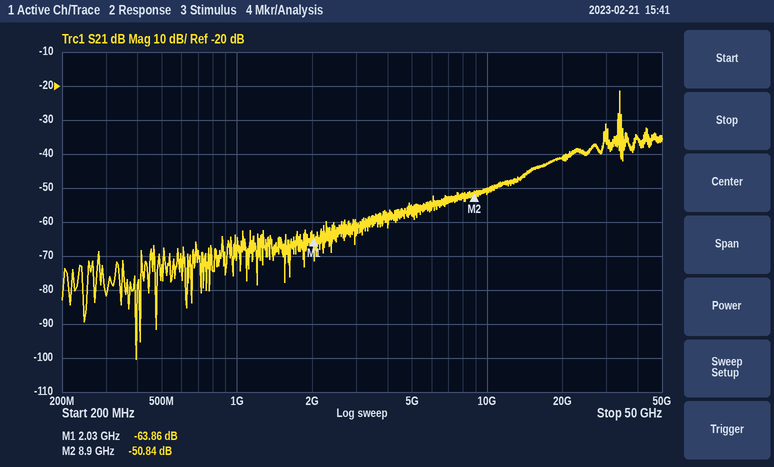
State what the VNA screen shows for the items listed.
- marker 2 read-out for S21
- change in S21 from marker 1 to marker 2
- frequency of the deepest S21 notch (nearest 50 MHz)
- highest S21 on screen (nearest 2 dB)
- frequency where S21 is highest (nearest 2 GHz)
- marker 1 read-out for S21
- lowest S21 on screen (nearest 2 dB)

-50.84 dB
13.02 dB
400 MHz
-22 dB
34 GHz
-63.86 dB
-100 dB
